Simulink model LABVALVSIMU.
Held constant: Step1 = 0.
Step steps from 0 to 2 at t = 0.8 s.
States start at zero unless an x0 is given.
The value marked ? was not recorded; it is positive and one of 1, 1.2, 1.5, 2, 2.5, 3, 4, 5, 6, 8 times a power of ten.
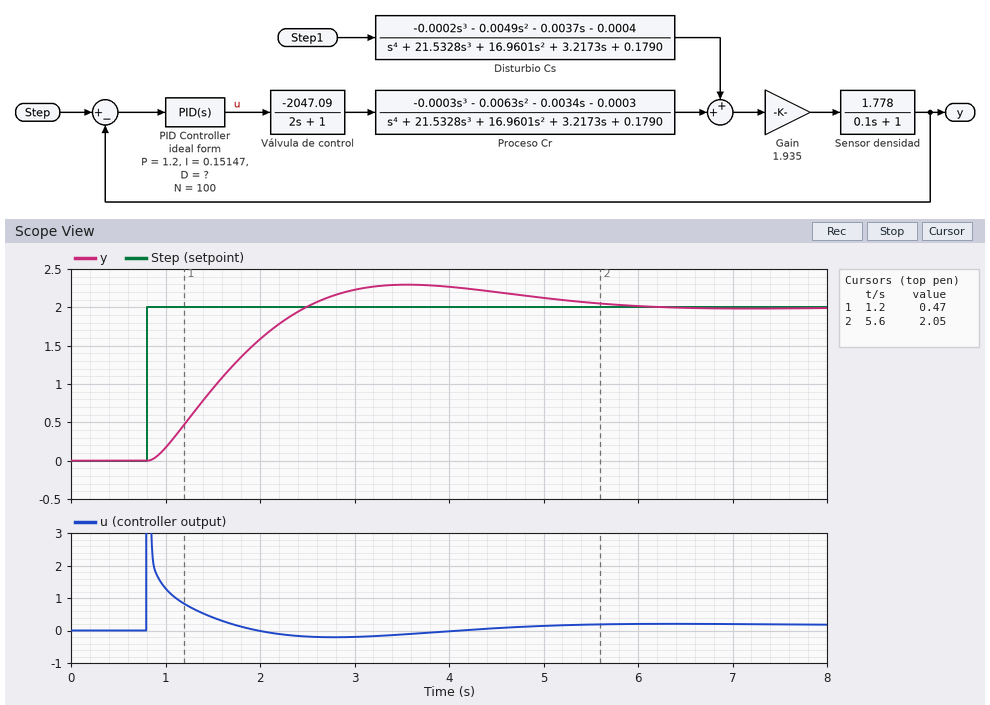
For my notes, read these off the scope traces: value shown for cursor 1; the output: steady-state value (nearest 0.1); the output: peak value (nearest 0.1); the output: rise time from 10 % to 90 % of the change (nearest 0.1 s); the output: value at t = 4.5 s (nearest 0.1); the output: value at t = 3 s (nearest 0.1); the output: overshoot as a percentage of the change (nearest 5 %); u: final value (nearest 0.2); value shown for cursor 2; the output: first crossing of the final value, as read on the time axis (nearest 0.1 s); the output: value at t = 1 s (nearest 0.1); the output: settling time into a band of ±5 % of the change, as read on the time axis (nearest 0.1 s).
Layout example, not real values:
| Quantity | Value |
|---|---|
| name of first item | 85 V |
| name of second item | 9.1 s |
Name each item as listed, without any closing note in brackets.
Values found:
| Quantity | Value |
|---|---|
| value shown for cursor 1 | 0.47 |
| the output: steady-state value | 2.0 |
| the output: peak value | 2.3 |
| the output: rise time from 10 % to 90 % of the change | 1.2 s |
| the output: value at t = 4.5 s | 2.2 |
| the output: value at t = 3 s | 2.2 |
| the output: overshoot as a percentage of the change | 15 % |
| u: final value | 0.2 |
| value shown for cursor 2 | 2.05 |
| the output: first crossing of the final value, as read on the time axis | 2.5 s |
| the output: value at t = 1 s | 0.2 |
| the output: settling time into a band of ±5 % of the change, as read on the time axis | 5.2 s |
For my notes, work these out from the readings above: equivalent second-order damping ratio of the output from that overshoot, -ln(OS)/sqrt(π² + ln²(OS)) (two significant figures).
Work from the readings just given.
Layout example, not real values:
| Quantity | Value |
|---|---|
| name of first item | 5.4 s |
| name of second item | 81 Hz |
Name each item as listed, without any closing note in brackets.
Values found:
| Quantity | Value |
|---|---|
| equivalent second-order damping ratio of the output from that overshoot, -ln(OS)/sqrt(π² + ln²(OS)) | 0.52 |
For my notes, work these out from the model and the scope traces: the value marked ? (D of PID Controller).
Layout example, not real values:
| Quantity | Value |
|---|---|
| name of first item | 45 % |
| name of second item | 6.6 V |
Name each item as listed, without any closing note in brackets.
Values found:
| Quantity | Value |
|---|---|
| the value marked ? | 0.6 |
